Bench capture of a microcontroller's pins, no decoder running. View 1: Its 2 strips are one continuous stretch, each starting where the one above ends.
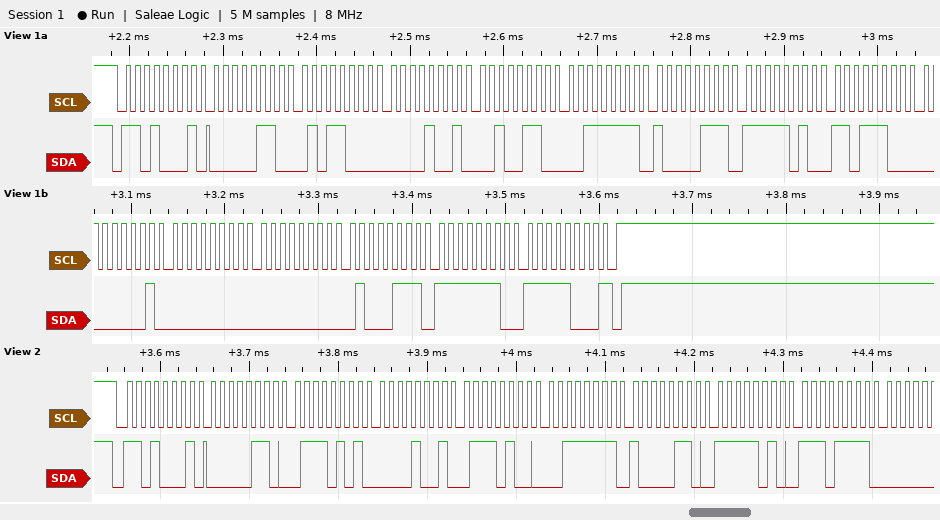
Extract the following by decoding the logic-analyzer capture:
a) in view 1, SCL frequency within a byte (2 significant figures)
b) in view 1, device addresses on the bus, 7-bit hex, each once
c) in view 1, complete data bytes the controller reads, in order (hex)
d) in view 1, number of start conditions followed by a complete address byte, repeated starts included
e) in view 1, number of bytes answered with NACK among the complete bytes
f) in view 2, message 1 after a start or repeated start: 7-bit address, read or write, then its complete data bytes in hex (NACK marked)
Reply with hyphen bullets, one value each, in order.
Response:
- 100 kHz
- 0x68
- 06 58 09 26 3F 87 FA DC 01 00 00 47 FE F8
- 1
- 1
- 0x68 read: 06 75 09 74 3F 86 FA EF
